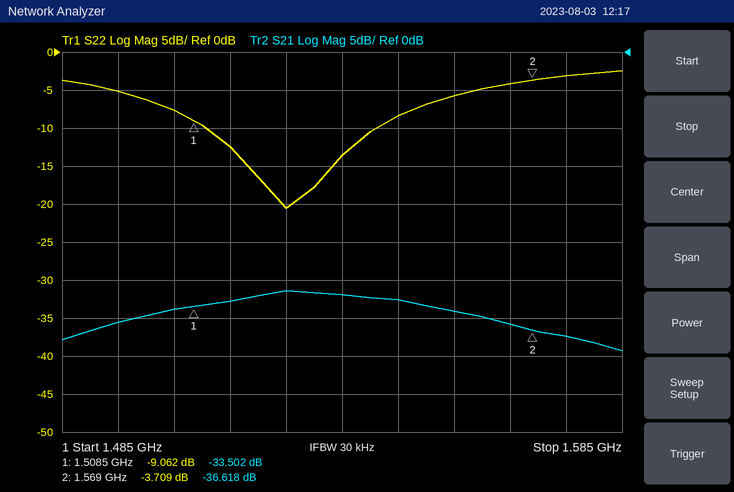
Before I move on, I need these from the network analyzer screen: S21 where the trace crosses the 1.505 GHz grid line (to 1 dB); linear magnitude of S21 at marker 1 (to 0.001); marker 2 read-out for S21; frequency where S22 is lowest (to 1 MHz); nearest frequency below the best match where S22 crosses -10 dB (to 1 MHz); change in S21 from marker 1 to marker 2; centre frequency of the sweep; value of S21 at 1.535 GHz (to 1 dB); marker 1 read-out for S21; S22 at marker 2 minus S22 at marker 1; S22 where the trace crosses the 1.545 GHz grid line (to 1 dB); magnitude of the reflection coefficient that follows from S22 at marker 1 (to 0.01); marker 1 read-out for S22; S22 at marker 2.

-34 dB
0.021
-36.618 dB
1.525 GHz
1.511 GHz
-3.116 dB
1.535 GHz
-32 dB
-33.502 dB
5.353 dB
-8 dB
0.35
-9.062 dB
-3.709 dB
